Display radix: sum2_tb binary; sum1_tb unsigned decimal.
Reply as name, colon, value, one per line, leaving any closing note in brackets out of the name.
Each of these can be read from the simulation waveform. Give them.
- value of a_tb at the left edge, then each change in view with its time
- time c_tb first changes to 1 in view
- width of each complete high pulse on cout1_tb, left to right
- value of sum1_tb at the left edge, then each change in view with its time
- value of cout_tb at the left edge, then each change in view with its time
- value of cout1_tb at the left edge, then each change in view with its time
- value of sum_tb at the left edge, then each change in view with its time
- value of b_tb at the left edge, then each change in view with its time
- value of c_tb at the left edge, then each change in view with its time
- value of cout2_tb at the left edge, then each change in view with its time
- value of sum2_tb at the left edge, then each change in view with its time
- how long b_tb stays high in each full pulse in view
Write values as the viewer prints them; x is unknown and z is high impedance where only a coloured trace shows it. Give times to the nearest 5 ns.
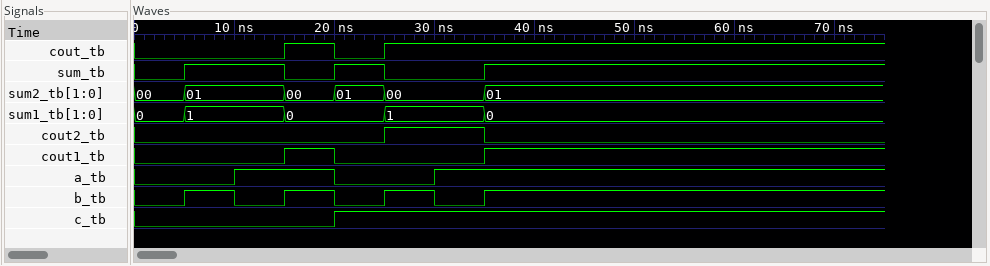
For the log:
value of a_tb at the left edge, then each change in view with its time: 0, 1 at 10 ns, 0 at 20 ns, 1 at 30 ns
time c_tb first changes to 1 in view: 20 ns
width of each complete high pulse on cout1_tb, left to right: 5 ns
value of sum1_tb at the left edge, then each change in view with its time: 0, 1 at 5 ns, 0 at 15 ns, 1 at 25 ns, 0 at 35 ns
value of cout_tb at the left edge, then each change in view with its time: 0, 1 at 15 ns, 0 at 20 ns, 1 at 25 ns
value of cout1_tb at the left edge, then each change in view with its time: 0, 1 at 15 ns, 0 at 20 ns, 1 at 35 ns
value of sum_tb at the left edge, then each change in view with its time: 0, 1 at 5 ns, 0 at 15 ns, 1 at 20 ns, 0 at 25 ns, 1 at 35 ns
value of b_tb at the left edge, then each change in view with its time: 0, 1 at 5 ns, 0 at 10 ns, 1 at 15 ns, 0 at 20 ns, 1 at 25 ns, 0 at 30 ns, 1 at 35 ns
value of c_tb at the left edge, then each change in view with its time: 0, 1 at 20 ns
value of cout2_tb at the left edge, then each change in view with its time: 0, 1 at 25 ns, 0 at 35 ns
value of sum2_tb at the left edge, then each change in view with its time: 00, 01 at 5 ns, 00 at 15 ns, 01 at 20 ns, 00 at 25 ns, 01 at 35 ns
how long b_tb stays high in each full pulse in view: 5 ns, 5 ns, 5 ns
